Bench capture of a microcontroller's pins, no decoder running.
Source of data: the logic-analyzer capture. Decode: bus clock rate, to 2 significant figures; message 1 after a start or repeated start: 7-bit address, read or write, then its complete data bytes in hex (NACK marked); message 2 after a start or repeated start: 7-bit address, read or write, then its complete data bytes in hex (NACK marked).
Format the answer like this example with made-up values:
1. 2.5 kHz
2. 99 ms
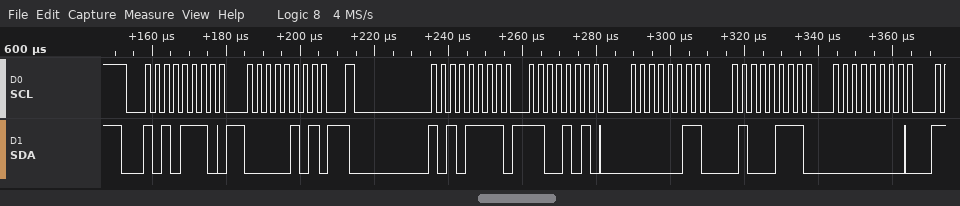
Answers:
1. 400 kHz
2. 0x57 write: 05
3. 0x57 read: CA 03 47 00
